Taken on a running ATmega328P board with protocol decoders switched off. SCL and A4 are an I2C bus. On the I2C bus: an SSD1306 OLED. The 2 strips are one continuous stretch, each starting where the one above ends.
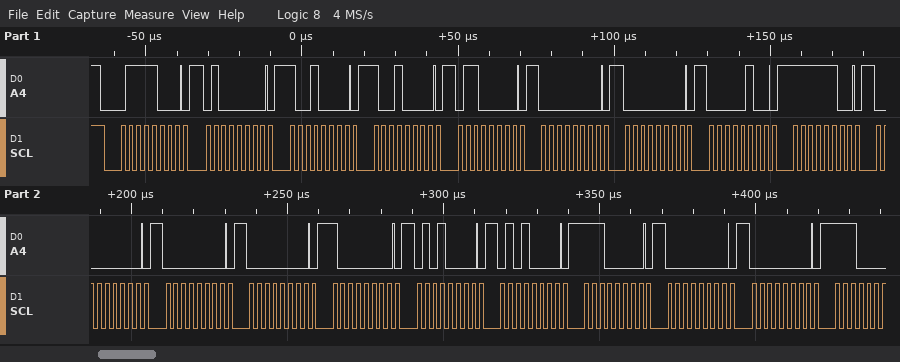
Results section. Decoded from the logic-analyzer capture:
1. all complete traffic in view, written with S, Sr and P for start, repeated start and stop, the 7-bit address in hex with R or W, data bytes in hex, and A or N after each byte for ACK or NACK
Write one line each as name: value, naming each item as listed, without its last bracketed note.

all complete traffic in view, written with S, Sr and P for start, repeated start and stop, the 7-bit address in hex with R or W, data bytes in hex, and A or N after each byte for ACK or NACK: S 3CW A 40 A 90 A 90 A 60 A 00 A 00 A 04 A FC A 00 A 00 A 00 A 80 A 50 A 50 A E0 A 00 A 00 A
